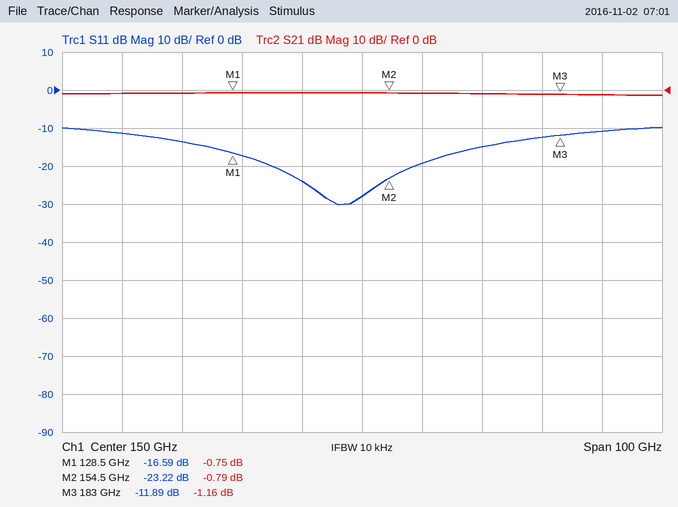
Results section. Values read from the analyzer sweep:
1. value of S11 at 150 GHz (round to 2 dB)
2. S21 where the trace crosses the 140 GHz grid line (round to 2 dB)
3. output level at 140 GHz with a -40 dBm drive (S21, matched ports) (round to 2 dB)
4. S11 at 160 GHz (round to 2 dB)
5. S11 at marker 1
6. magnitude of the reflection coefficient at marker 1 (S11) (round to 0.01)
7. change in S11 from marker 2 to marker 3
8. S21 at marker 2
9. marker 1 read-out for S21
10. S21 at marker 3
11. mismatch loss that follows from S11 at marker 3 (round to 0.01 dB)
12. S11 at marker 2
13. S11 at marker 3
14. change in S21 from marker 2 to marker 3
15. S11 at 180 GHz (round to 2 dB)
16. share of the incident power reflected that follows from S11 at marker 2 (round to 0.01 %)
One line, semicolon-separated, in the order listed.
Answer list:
-28 dB; 0 dB; -40 dBm; -20 dB; -16.59 dB; 0.15; 11.33 dB; -0.79 dB; -0.75 dB; -1.16 dB; 0.29 dB; -23.22 dB; -11.89 dB; -0.37 dB; -12 dB; 0.48 %
